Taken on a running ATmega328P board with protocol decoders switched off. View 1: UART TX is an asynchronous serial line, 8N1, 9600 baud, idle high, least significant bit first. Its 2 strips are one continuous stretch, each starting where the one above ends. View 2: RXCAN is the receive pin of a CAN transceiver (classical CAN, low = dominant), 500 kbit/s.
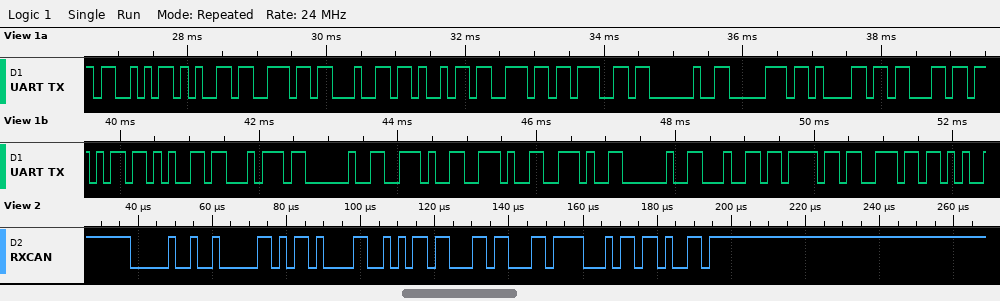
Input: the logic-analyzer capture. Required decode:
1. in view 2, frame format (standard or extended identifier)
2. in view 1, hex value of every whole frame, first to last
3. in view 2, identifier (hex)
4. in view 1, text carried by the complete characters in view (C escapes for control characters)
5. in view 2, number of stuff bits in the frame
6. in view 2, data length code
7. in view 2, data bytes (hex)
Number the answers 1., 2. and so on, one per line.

1. standard
2. 53 65 6E 64 69 6E 67 20 70 61 63 6B 65 74 20 2E 2E 2E 20 64 6F 6E
3. 0x012
4. "Sending packet ... don"
5. 2
6. 5
7. 68 65 6C 6C 6F
